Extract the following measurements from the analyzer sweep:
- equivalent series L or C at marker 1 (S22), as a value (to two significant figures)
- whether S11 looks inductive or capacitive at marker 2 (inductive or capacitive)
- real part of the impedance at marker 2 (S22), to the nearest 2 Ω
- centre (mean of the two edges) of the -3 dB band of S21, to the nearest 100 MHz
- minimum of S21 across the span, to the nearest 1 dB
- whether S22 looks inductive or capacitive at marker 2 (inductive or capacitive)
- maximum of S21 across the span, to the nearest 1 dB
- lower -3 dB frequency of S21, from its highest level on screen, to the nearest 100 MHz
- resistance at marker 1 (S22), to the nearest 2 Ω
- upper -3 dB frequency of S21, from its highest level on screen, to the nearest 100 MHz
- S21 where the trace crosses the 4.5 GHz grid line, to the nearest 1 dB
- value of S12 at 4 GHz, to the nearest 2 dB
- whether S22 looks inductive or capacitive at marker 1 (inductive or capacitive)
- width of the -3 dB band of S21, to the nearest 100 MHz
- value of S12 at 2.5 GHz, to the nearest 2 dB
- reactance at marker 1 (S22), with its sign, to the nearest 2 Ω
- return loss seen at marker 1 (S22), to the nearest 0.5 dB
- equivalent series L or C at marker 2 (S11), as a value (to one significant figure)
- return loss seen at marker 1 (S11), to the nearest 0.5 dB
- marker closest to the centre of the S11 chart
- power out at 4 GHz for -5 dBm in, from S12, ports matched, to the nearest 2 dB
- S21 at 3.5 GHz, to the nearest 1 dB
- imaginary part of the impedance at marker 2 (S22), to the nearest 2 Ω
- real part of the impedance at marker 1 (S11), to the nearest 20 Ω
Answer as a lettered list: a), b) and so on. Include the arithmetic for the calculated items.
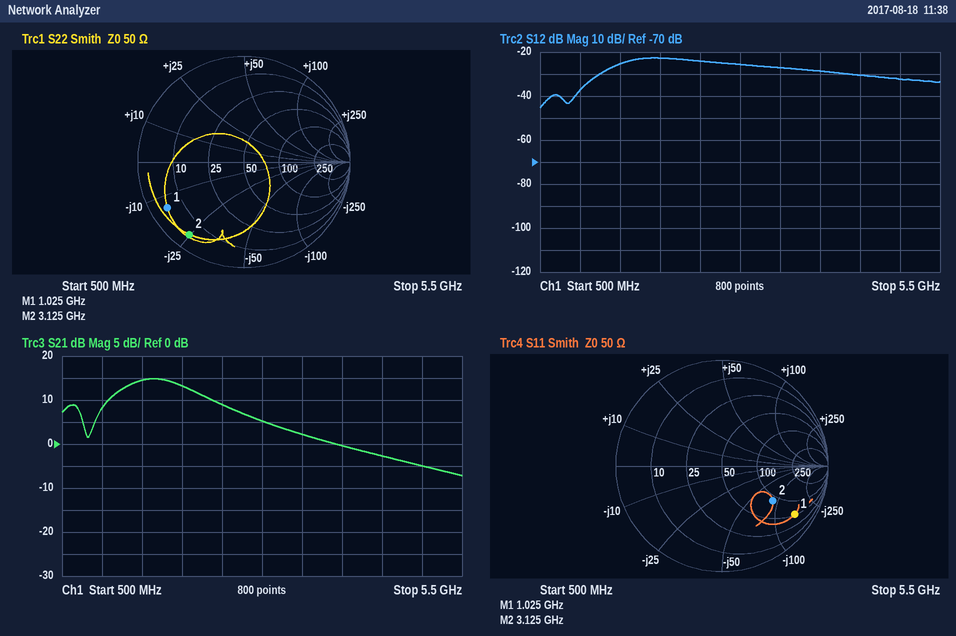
a) C = 1/(2π × 1.025 GHz × 14 Ω) ≈ 11 pF
b) capacitive
c) 4 Ω
d) 1.7 GHz
e) -7 dB
f) capacitive
g) 15 dB
h) 1.2 GHz
i) 4 Ω
j) 2.2 GHz
k) -3 dB
l) -28 dB
m) capacitive
n) 2.2 GHz − 1.2 GHz = 1.0 GHz
o) -24 dB
p) -14 Ω
q) 1.5 dB
r) C = 1/(2π × 3.125 GHz × 90 Ω) ≈ 566 fF, so 600 fF to one significant figure
s) 1.5 dB
t) marker 2
u) -5 dBm + (-28 dB) = -34 dBm
v) 2 dB
w) -24 Ω
x) 60 Ω
